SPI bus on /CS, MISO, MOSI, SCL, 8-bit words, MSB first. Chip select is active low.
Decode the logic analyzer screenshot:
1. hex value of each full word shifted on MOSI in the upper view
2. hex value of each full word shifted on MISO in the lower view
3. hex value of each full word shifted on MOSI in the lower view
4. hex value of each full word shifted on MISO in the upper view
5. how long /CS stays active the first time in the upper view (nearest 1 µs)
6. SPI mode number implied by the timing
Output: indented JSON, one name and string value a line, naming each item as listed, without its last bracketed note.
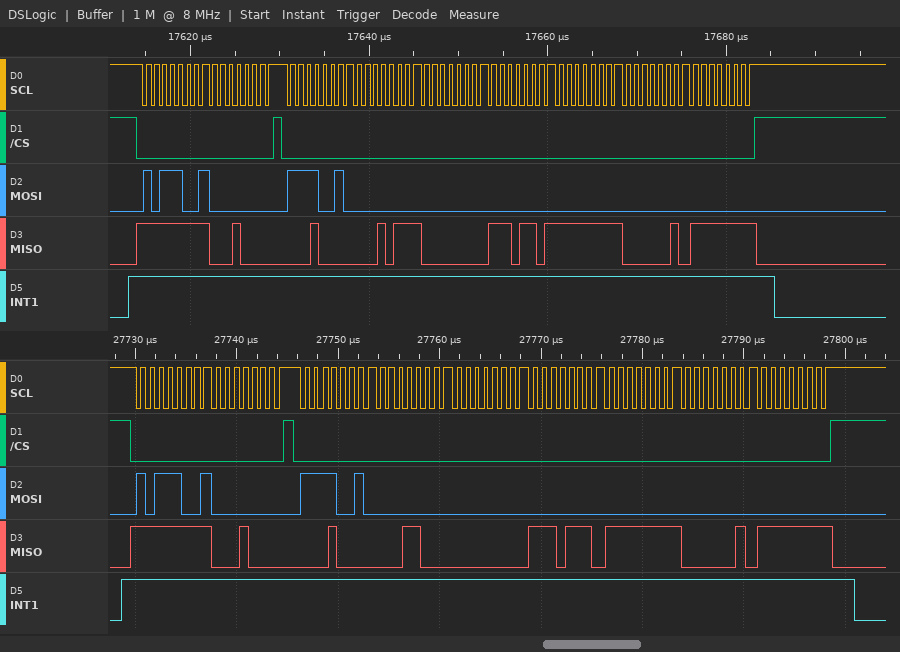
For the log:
{
  "hex value of each full word shifted on MOSI in the upper view": "B9, 00, F2, 00, 00, 00, 00, 00, 00",
  "hex value of each full word shifted on MISO in the lower view": "FF, 10, 10, 18, 00, EE, FF, 02, FF",
  "hex value of each full word shifted on MOSI in the lower view": "B9, 00, F2, 00, 00, 00, 00, 00, 00",
  "hex value of each full word shifted on MISO in the upper view": "FF, 10, 10, 17, 00, ED, FF, 02, FF",
  "how long /CS stays active the first time in the upper view": "15 µs",
  "SPI mode number implied by the timing": "3"
}
